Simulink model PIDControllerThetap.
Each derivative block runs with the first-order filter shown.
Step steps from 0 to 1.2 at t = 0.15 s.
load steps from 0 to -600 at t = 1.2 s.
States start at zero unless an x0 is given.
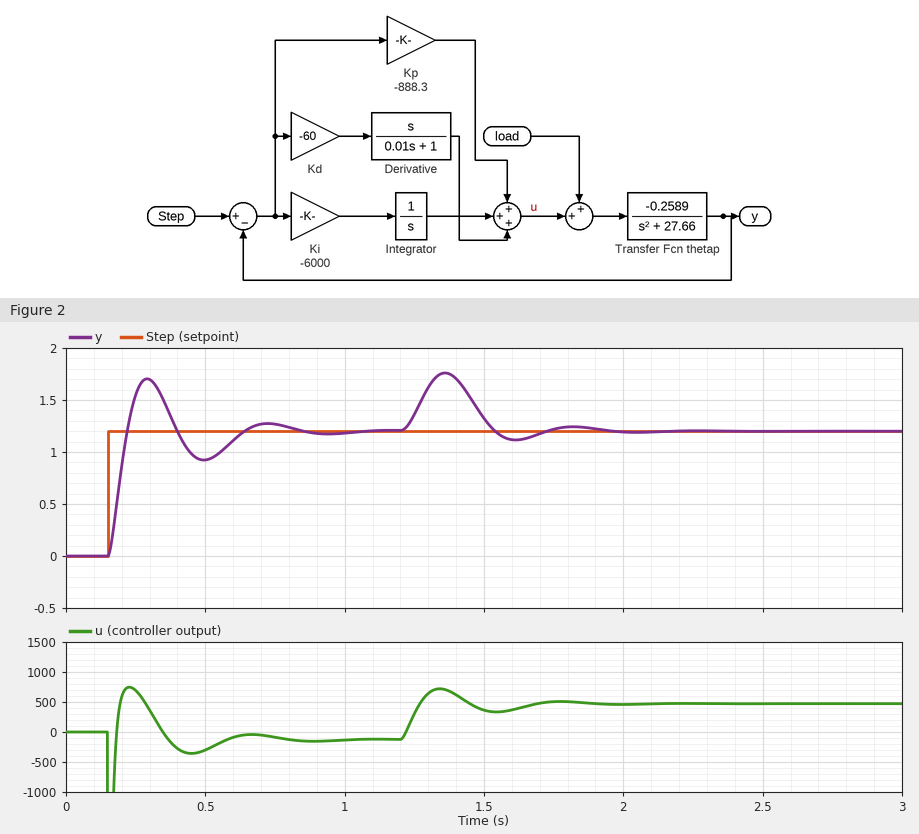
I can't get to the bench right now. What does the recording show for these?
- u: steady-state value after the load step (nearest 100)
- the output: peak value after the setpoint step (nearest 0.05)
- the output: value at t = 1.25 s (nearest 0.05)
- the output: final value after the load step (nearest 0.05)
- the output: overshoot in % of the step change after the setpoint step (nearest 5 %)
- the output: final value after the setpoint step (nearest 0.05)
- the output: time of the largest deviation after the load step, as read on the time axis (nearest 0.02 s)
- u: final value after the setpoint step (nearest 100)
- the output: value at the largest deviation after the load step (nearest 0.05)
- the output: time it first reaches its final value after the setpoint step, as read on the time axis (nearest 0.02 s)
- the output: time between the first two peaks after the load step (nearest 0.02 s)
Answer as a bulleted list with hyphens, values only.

- 500
- 1.70
- 1.35
- 1.20
- 40 %
- 1.20
- 1.36 s
- -100
- 1.75
- 0.22 s
- 0.46 s
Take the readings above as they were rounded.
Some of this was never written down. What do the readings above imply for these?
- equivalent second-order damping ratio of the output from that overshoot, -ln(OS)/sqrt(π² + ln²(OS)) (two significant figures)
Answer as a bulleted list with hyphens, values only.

- 0.28
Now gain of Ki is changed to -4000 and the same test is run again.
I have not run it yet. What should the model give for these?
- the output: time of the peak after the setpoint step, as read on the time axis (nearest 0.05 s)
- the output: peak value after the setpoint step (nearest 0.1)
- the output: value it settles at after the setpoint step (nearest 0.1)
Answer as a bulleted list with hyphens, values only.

- 0.30 s
- 1.6
- 1.2
